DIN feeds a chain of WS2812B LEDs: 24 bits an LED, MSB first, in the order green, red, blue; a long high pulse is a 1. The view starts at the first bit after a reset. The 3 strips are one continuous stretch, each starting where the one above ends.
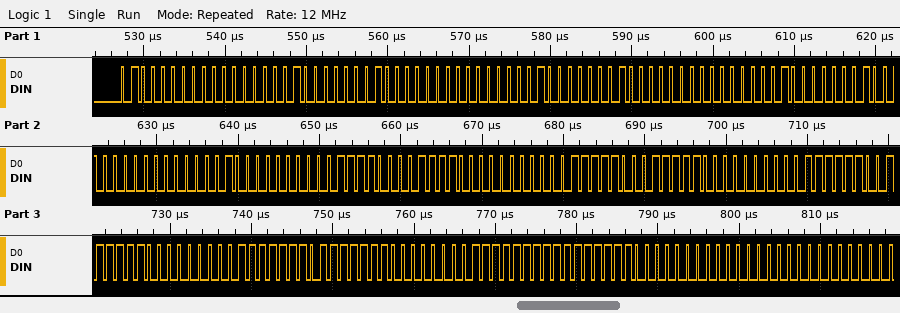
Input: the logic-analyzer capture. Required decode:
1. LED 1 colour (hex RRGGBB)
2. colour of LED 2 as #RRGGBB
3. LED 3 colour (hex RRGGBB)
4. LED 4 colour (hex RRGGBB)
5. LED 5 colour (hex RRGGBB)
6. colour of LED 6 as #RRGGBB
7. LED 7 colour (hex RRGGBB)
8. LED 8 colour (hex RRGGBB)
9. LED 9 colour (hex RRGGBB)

#004040
#004040
#004040
#004040
#0F0F00
#1F1F00
#3F3F00
#7F7F00
#FFFF00
